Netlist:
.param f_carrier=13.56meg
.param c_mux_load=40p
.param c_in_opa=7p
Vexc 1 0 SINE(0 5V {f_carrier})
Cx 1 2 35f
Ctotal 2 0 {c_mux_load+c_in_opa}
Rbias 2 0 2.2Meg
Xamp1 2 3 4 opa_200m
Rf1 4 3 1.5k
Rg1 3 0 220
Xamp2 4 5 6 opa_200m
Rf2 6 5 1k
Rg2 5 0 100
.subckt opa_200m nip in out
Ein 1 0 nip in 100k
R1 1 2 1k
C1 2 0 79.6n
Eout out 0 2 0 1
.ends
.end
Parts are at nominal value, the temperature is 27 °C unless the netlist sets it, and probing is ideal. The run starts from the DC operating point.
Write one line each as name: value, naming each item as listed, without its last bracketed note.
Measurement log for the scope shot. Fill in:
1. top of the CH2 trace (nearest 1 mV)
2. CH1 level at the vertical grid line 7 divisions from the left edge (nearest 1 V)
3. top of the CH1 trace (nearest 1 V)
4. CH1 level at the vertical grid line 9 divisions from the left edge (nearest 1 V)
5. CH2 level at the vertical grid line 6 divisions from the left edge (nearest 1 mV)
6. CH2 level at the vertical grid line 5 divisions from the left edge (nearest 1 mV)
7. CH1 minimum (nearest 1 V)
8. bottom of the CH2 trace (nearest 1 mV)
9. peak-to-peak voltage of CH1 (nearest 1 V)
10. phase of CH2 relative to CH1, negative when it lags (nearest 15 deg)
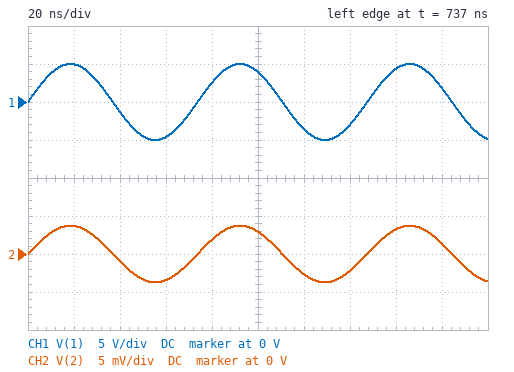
top of the CH2 trace: 4 mV
CH1 level at the vertical grid line 7 divisions from the left edge: -3 V
top of the CH1 trace: 5 V
CH1 level at the vertical grid line 9 divisions from the left edge: 2 V
CH2 level at the vertical grid line 6 divisions from the left edge: -3 mV
CH2 level at the vertical grid line 5 divisions from the left edge: 3 mV
CH1 minimum: -5 V
bottom of the CH2 trace: -4 mV
peak-to-peak voltage of CH1: 10 V
phase of CH2 relative to CH1, negative when it lags: 0 deg
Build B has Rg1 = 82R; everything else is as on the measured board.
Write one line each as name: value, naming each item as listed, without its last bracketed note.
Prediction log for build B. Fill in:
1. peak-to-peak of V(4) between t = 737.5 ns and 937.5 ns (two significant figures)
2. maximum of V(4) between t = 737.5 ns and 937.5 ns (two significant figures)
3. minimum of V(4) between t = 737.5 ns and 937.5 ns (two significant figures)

peak-to-peak of V(4) between t = 737.5 ns and 937.5 ns: 87 mV
maximum of V(4) between t = 737.5 ns and 937.5 ns: 44 mV
minimum of V(4) between t = 737.5 ns and 937.5 ns: -44 mV
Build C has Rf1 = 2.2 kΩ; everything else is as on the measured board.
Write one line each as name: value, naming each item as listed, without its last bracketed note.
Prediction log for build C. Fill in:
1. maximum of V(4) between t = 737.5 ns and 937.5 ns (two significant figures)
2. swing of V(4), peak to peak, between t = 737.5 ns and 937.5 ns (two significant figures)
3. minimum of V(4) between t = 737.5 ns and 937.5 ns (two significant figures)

maximum of V(4) between t = 737.5 ns and 937.5 ns: 33 mV
swing of V(4), peak to peak, between t = 737.5 ns and 937.5 ns: 66 mV
minimum of V(4) between t = 737.5 ns and 937.5 ns: -33 mV
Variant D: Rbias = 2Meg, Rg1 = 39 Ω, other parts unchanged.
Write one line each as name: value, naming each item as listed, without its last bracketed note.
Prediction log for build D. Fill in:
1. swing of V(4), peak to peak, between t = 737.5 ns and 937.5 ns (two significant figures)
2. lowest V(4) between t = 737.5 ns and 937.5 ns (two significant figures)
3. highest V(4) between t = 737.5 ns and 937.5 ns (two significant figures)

swing of V(4), peak to peak, between t = 737.5 ns and 937.5 ns: 100 mV
lowest V(4) between t = 737.5 ns and 937.5 ns: -51 mV
highest V(4) between t = 737.5 ns and 937.5 ns: 51 mV
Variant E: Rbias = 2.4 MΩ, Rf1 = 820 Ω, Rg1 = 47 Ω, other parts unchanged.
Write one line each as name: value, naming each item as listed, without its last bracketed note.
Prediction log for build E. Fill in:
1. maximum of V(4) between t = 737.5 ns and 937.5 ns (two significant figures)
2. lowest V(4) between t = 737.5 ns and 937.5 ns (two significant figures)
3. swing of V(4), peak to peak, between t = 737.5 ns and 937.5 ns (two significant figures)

maximum of V(4) between t = 737.5 ns and 937.5 ns: 43 mV
lowest V(4) between t = 737.5 ns and 937.5 ns: -43 mV
swing of V(4), peak to peak, between t = 737.5 ns and 937.5 ns: 86 mV
